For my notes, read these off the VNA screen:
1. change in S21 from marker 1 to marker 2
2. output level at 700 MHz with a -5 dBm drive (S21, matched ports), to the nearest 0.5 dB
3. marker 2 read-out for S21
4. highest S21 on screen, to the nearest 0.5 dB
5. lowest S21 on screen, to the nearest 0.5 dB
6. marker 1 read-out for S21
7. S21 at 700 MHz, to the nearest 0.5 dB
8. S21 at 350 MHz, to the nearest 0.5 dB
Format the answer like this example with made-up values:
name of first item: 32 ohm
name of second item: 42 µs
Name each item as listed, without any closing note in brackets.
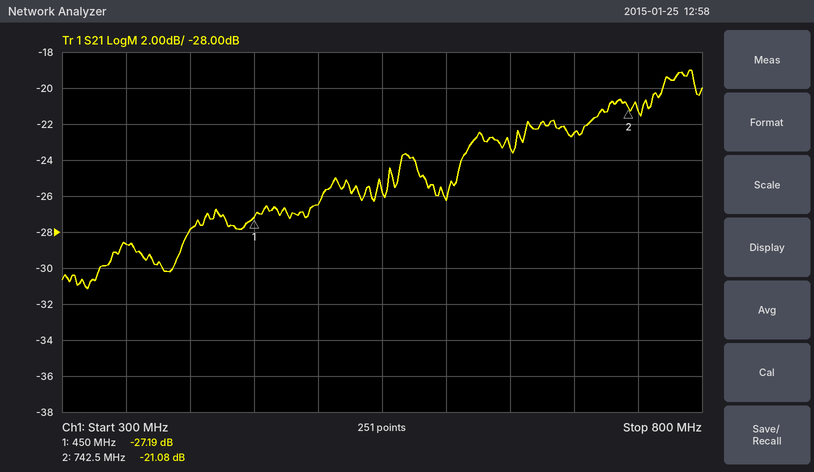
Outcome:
change in S21 from marker 1 to marker 2: 6.11 dB
output level at 700 MHz with a -5 dBm drive (S21, matched ports), to the nearest 0.5 dB: -27.5 dBm
marker 2 read-out for S21: -21.08 dB
highest S21 on screen, to the nearest 0.5 dB: -19.0 dB
lowest S21 on screen, to the nearest 0.5 dB: -31.0 dB
marker 1 read-out for S21: -27.19 dB
S21 at 700 MHz, to the nearest 0.5 dB: -22.5 dB
S21 at 350 MHz, to the nearest 0.5 dB: -28.5 dB
